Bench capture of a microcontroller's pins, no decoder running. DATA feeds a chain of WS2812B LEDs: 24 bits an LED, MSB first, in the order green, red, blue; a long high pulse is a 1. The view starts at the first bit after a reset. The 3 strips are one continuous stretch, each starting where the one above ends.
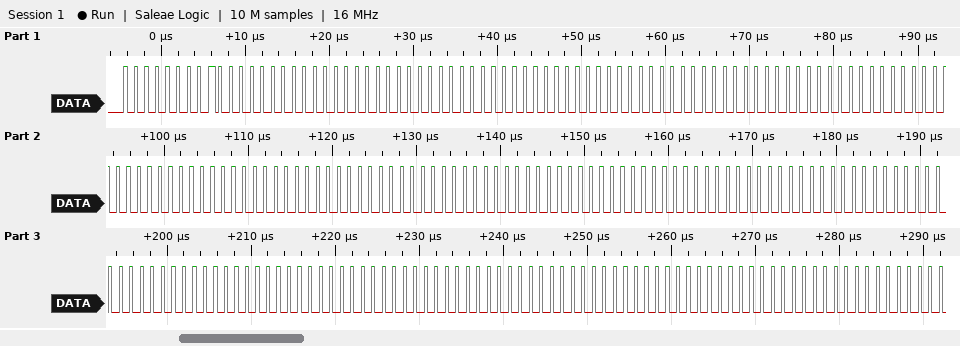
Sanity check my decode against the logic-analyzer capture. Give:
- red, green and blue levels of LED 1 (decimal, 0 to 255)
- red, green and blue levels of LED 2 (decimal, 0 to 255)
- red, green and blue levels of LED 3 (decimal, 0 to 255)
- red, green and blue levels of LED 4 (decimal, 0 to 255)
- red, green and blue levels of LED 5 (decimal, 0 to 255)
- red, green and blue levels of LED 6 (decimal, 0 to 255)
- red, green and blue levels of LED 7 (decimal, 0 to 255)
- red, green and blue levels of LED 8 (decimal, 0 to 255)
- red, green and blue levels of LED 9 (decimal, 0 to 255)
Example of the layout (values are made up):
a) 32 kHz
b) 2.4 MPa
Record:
a) 128, 0, 0
b) 0, 0, 0
c) 0, 0, 0
d) 0, 0, 0
e) 0, 0, 0
f) 0, 0, 0
g) 0, 0, 0
h) 0, 0, 0
i) 0, 0, 0
